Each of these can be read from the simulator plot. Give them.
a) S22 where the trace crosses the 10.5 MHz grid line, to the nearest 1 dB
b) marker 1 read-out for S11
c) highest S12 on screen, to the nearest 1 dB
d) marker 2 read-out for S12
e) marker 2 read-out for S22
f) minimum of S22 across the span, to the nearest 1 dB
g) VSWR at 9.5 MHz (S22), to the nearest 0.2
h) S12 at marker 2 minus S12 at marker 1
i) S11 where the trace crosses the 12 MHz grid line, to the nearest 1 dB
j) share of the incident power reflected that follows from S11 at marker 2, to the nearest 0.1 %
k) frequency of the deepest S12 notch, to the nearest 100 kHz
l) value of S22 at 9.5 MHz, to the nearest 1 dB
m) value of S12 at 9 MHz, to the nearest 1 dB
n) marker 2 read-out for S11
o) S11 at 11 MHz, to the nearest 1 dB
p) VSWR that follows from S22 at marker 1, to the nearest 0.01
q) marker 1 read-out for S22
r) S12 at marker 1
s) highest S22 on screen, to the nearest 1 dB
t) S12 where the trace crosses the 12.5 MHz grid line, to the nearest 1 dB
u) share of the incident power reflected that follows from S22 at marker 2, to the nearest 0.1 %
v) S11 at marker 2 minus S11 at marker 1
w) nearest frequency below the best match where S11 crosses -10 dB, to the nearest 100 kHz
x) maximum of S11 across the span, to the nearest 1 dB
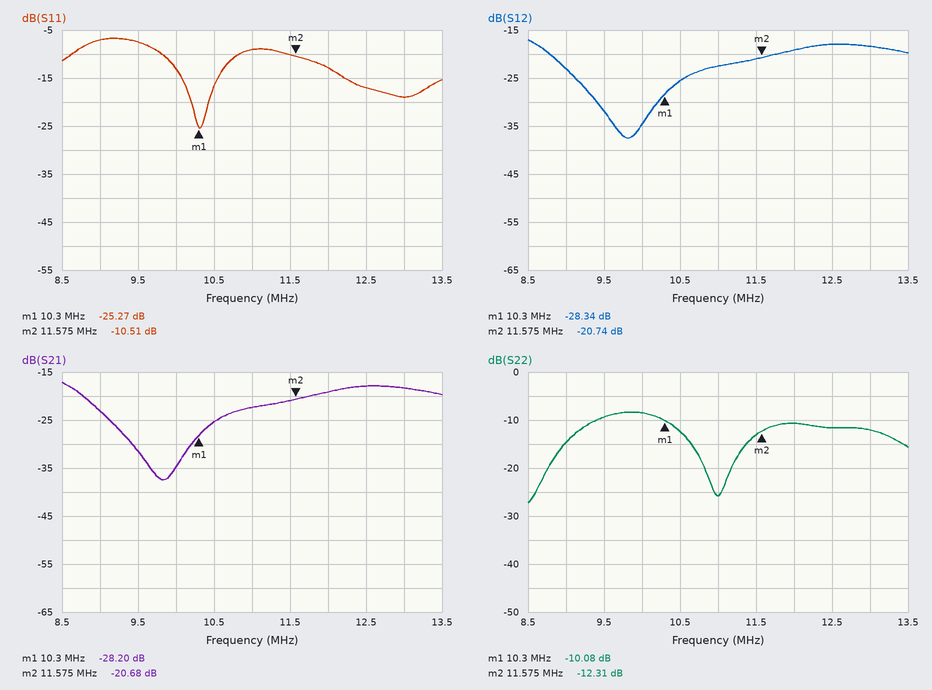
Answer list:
-12 dB
-25.27 dB
-17 dB
-20.74 dB
-12.31 dB
-27 dB
2.0
7.60 dB
-13 dB
8.9 %
9.8 MHz
-9 dB
-23 dB
-10.51 dB
-9 dB
1.91
-10.08 dB
-28.34 dB
-8 dB
-18 dB
5.9 %
14.76 dB
9.8 MHz
-7 dB
